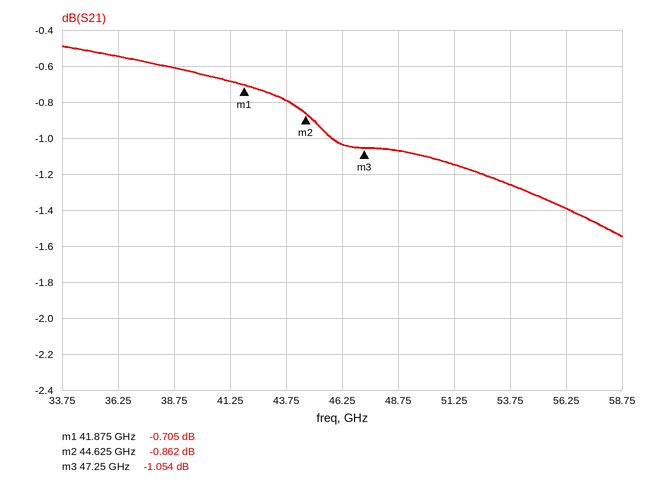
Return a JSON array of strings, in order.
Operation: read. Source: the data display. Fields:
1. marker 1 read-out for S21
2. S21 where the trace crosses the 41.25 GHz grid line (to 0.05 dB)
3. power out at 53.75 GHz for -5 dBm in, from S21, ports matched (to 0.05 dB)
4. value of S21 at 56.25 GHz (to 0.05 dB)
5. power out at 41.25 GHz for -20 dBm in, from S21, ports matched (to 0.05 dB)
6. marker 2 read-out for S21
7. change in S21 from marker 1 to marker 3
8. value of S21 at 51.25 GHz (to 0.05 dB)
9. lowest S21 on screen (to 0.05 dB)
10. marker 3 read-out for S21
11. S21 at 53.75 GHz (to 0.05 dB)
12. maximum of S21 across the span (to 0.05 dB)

["-0.705 dB", "-0.70 dB", "-6.25 dBm", "-1.40 dB", "-20.70 dBm", "-0.862 dB", "-0.349 dB", "-1.15 dB", "-1.55 dB", "-1.054 dB", "-1.25 dB", "-0.50 dB"]
